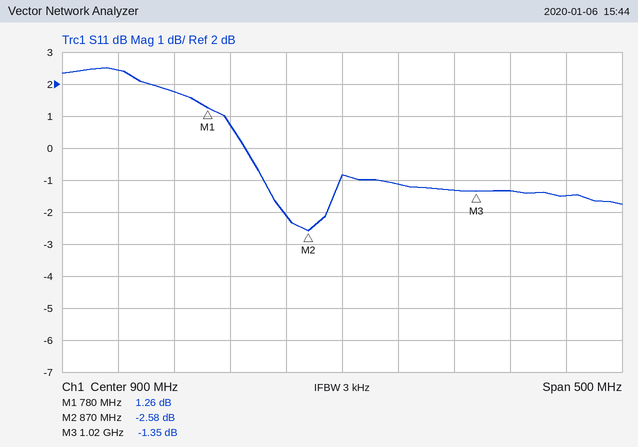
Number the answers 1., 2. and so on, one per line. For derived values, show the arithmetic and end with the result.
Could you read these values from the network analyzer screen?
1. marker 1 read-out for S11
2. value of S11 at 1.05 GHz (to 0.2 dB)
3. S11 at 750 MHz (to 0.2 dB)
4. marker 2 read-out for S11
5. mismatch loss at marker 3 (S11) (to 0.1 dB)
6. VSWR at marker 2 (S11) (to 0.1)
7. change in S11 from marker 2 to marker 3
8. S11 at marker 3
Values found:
1. 1.26 dB
2. -1.4 dB
3. 1.8 dB
4. -2.58 dB
5. −10 log10(1 − 10^(-1.35/10)) ≈ 5.7 dB
6. (1 + 0.7430)/(1 − 0.7430) ≈ 6.8
7. -1.35 − (-2.58) = 1.23 dB
8. -1.35 dB
